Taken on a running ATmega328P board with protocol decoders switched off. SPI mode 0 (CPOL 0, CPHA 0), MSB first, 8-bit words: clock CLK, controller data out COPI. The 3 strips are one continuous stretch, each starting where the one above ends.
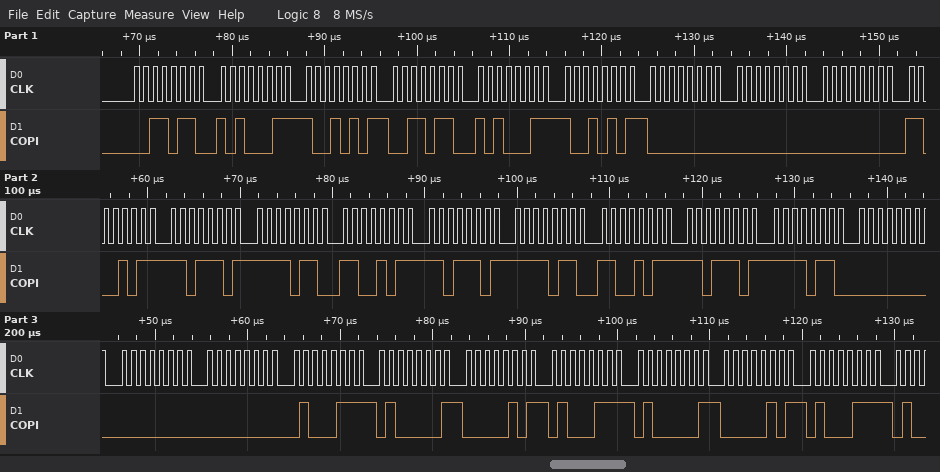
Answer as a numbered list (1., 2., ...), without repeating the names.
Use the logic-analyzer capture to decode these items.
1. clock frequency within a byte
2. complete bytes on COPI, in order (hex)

1. 1 MHz
2. 0x36 0xA3 0x95 0x36 0xA3 0x95 0x00 0x00 0x00 0xCB 0xDD 0xF6 0xCB 0xDD 0xF6 0xCB 0xDD 0xF6 0x00 0x00 0x00 0x47 0x41 0x05 0x47 0x41 0x05 0x47
